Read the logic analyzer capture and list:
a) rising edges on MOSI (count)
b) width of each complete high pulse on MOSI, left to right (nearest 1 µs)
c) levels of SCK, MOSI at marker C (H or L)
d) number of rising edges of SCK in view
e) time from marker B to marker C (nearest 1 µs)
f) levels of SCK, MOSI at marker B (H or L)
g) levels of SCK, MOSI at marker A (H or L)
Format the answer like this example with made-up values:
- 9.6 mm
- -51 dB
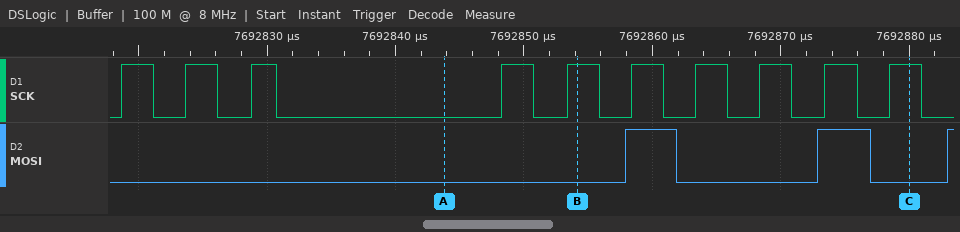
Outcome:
- 3
- 4 µs, 4 µs
- SCK=H, MOSI=L
- 10
- 26 µs
- SCK=H, MOSI=L
- SCK=L, MOSI=L
